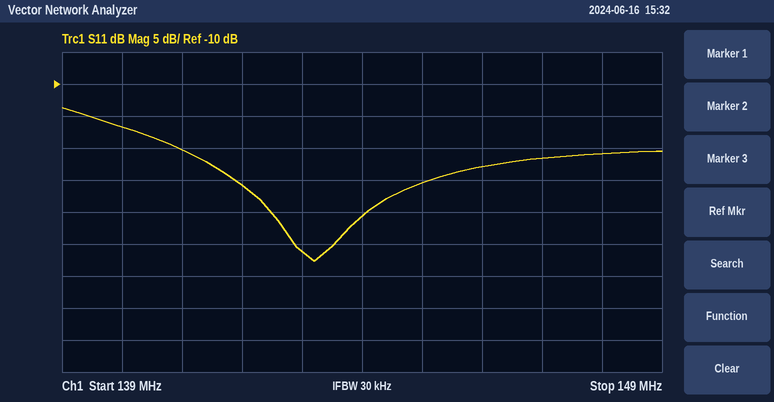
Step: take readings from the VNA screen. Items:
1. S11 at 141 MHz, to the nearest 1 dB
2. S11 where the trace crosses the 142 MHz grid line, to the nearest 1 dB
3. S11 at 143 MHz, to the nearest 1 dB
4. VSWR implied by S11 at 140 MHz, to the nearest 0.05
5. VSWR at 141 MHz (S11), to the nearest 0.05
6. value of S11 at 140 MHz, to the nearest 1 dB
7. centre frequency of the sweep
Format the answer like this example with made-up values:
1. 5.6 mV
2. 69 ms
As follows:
1. -20 dB
2. -26 dB
3. -36 dB
4. 1.35
5. 1.20
6. -17 dB
7. 144 MHz
